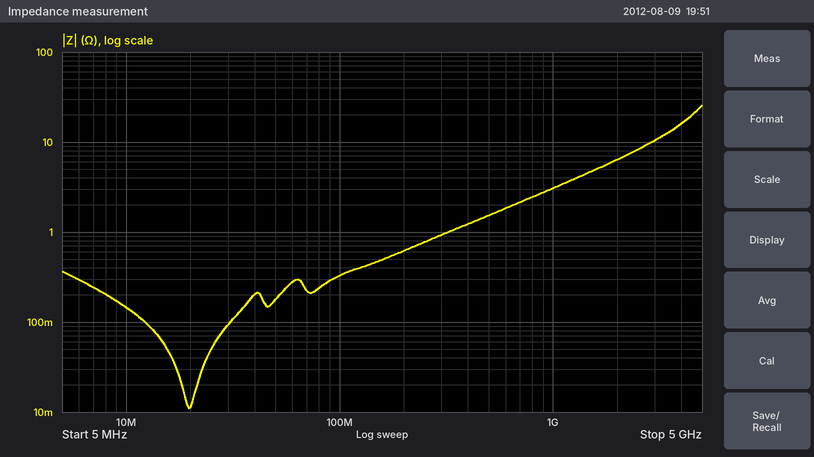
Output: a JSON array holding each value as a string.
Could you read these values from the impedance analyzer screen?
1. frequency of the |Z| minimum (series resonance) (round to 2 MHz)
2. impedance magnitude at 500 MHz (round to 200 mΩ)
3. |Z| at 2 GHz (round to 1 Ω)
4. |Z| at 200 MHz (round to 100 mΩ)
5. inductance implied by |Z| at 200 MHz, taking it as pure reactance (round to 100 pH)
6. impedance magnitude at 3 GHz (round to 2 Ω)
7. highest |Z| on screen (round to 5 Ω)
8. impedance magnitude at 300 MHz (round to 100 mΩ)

["20 MHz", "1.6 Ω", "6 Ω", "600 mΩ", "500 pH", "10 Ω", "25 Ω", "900 mΩ"]
